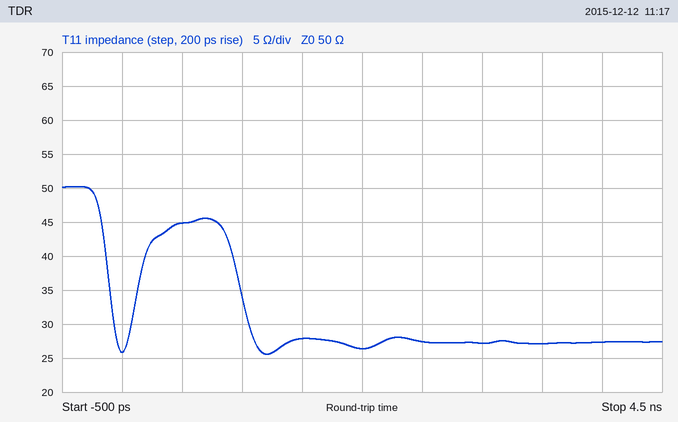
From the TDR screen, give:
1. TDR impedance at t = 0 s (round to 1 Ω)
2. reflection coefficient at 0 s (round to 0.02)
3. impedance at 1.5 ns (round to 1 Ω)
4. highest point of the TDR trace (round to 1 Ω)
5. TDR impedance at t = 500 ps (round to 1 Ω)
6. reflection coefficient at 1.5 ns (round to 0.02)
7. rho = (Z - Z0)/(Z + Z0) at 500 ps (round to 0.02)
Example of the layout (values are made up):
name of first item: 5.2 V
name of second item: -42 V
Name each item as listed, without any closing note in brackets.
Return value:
TDR impedance at t = 0 s: 26 Ω
reflection coefficient at 0 s: -0.32
impedance at 1.5 ns: 28 Ω
highest point of the TDR trace: 50 Ω
TDR impedance at t = 500 ps: 45 Ω
reflection coefficient at 1.5 ns: -0.28
rho = (Z - Z0)/(Z + Z0) at 500 ps: -0.06
